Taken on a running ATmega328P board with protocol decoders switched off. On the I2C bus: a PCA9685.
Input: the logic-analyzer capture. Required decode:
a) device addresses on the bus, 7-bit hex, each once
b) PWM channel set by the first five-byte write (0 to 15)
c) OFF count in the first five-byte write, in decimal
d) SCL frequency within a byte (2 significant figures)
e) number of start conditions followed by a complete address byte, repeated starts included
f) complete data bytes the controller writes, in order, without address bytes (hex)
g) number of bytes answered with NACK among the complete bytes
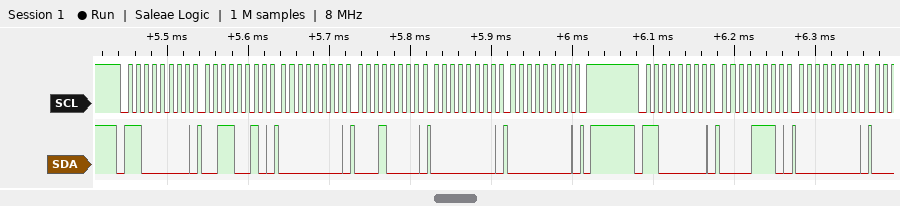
0x60
11
0
100 kHz
2
32 00 10 00 00 0E 00
0
